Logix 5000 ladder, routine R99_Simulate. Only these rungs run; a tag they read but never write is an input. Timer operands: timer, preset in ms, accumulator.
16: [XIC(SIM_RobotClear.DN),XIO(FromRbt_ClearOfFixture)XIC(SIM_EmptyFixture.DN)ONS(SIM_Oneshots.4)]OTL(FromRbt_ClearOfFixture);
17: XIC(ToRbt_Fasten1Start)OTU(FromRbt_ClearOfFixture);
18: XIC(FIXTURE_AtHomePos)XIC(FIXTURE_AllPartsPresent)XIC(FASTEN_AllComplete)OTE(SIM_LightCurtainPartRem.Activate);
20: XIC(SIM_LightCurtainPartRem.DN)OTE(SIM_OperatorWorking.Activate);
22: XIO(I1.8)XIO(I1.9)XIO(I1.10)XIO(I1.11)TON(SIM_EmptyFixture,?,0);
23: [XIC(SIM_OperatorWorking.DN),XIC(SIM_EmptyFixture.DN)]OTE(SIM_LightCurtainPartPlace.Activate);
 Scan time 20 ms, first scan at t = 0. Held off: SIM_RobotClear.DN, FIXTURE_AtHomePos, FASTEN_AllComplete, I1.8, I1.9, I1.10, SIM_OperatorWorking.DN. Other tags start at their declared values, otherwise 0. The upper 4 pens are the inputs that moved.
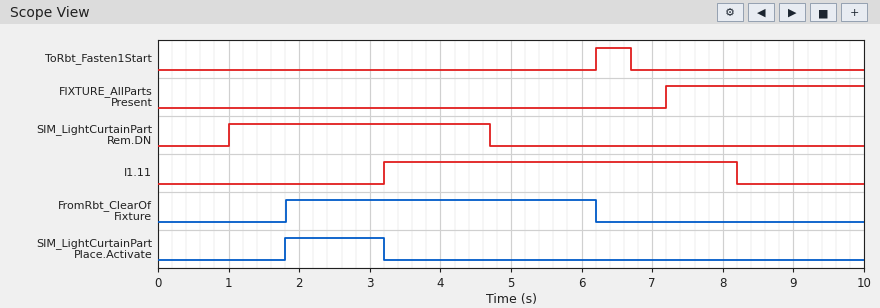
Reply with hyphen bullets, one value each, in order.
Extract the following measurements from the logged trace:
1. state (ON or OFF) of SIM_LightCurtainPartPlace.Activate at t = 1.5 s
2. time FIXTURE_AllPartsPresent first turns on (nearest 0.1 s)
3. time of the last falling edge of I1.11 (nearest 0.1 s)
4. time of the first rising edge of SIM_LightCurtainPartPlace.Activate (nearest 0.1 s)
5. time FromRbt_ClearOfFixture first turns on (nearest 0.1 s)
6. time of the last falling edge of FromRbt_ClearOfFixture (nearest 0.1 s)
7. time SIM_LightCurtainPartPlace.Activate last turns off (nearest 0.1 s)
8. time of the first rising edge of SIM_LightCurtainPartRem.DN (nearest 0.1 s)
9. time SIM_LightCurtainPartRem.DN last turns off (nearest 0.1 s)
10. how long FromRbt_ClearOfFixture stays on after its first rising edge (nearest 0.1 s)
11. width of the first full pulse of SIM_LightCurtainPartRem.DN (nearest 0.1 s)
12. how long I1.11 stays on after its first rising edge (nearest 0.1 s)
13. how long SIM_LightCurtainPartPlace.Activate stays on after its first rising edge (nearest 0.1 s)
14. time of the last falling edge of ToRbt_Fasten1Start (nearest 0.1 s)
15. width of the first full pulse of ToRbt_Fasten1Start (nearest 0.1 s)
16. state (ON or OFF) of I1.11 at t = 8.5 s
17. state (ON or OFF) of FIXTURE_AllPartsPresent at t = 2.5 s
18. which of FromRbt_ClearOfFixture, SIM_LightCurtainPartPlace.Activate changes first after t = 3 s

- OFF
- 7.2 s
- 8.2 s
- 1.8 s
- 1.8 s
- 6.2 s
- 3.2 s
- 1.0 s
- 4.7 s
- 4.4 s
- 3.7 s
- 5.0 s
- 1.4 s
- 6.7 s
- 0.5 s
- OFF
- OFF
- SIM_LightCurtainPartPlace.Activate
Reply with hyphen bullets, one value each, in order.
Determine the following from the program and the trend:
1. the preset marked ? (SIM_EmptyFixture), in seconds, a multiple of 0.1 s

- 1.8 s
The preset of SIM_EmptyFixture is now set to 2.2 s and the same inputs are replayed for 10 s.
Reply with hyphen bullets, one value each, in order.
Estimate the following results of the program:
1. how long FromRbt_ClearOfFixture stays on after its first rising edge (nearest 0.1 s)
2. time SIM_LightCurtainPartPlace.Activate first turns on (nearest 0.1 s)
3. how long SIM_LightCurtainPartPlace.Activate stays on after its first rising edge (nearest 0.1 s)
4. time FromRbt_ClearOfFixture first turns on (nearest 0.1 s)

- 4.0 s
- 2.2 s
- 1.0 s
- 2.2 s
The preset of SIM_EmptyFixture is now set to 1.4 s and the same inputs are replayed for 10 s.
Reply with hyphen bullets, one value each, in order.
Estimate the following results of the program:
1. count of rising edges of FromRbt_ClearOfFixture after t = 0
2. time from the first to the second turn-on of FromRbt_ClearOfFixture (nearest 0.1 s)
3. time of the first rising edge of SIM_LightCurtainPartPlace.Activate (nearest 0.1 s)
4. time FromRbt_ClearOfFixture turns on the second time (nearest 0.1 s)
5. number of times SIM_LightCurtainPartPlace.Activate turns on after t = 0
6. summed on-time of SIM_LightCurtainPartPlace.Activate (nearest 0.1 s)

- 2
- 8.2 s
- 1.4 s
- 9.6 s
- 2
- 2.2 s
